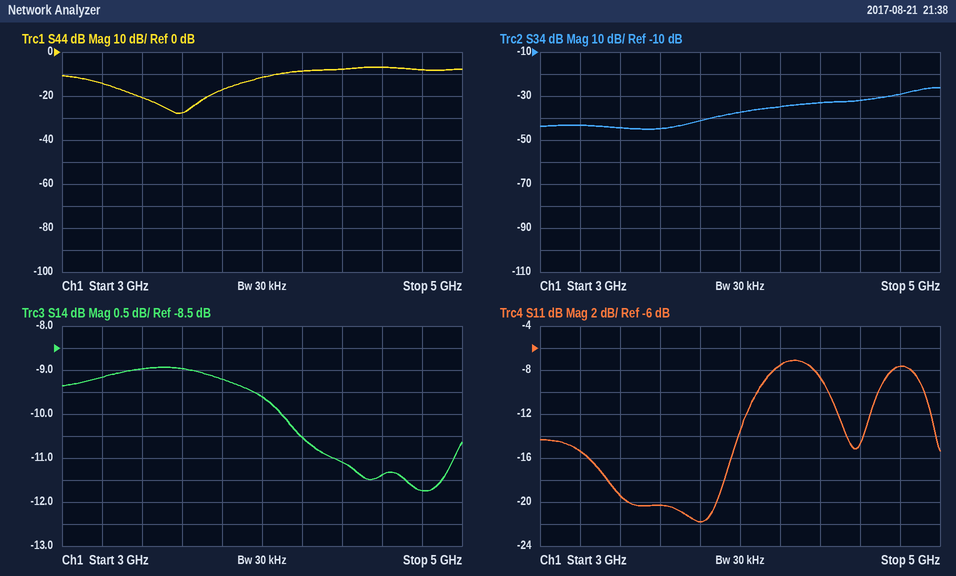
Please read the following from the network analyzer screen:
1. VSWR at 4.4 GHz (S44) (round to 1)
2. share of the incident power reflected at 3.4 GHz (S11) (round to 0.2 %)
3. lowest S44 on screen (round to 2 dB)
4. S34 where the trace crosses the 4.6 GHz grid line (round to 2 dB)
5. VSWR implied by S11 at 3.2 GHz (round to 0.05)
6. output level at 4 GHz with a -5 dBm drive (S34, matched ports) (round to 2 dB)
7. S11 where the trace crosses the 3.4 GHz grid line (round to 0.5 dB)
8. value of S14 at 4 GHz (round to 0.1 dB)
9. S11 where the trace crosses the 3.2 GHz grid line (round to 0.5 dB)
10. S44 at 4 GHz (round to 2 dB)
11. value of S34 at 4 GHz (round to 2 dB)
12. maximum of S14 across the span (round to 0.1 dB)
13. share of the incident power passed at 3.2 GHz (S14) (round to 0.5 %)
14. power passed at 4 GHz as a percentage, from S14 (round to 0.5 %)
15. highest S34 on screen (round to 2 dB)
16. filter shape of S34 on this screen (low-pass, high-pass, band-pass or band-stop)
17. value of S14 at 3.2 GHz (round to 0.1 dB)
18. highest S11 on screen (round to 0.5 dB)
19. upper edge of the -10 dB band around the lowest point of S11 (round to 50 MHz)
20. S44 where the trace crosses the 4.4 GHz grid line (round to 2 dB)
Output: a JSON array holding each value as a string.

["2", "1.2 %", "-28 dB", "-32 dB", "1.40", "-42 dBm", "-19.5 dB", "-9.6 dB", "-15.5 dB", "-12 dB", "-38 dB", "-8.9 dB", "12.0 %", "11.0 %", "-26 dB", "high-pass", "-9.2 dB", "-7.0 dB", "4.10 GHz", "-8 dB"]
